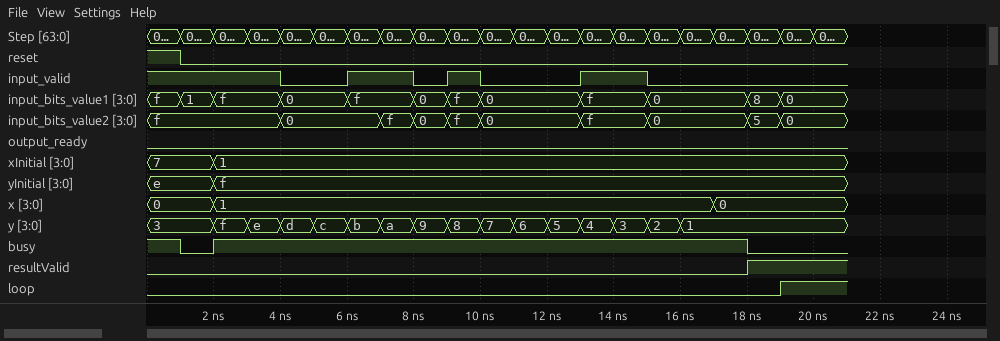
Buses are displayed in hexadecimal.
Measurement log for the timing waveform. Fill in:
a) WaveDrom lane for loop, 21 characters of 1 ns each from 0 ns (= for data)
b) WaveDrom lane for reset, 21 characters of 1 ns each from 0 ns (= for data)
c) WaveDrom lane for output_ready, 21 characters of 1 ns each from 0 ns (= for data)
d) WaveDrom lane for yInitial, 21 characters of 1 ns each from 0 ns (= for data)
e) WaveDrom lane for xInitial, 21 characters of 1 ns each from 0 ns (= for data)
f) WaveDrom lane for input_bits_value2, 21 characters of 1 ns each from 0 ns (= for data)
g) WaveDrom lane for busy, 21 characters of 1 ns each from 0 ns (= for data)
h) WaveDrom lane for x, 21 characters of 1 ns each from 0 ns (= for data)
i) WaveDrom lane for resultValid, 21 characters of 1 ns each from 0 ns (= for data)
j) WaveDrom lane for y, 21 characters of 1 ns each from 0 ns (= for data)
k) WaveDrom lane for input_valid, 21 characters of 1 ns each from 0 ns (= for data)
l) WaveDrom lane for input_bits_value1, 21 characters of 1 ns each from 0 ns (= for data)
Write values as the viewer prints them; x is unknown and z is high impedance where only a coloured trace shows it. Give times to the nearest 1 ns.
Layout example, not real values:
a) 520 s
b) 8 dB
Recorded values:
a) {name: 'loop', wave: '0..................1.'}
b) {name: 'reset', wave: '10...................'}
c) {name: 'output_ready', wave: '0....................'}
d) {name: 'yInitial', wave: '=.=..................', data: 'e f'}
e) {name: 'xInitial', wave: '=.=..................', data: '7 1'}
f) {name: 'input_bits_value2', wave: '=...=..====..=.=..==.', data: 'f 0 f 0 f 0 f 0 5 0'}
g) {name: 'busy', wave: '101...............0..'}
h) {name: 'x', wave: '=.=..............=...', data: '0 1 0'}
i) {name: 'resultValid', wave: '0.................1..'}
j) {name: 'y', wave: '=.===============....', data: '3 f e d c b a 9 8 7 6 5 4 3 2 1'}
k) {name: 'input_valid', wave: '1...0.1.010..1.0.....'}
l) {name: 'input_bits_value1', wave: '===.=.=.===..=.=..==.', data: 'f 1 f 0 f 0 f 0 f 0 8 0'}
